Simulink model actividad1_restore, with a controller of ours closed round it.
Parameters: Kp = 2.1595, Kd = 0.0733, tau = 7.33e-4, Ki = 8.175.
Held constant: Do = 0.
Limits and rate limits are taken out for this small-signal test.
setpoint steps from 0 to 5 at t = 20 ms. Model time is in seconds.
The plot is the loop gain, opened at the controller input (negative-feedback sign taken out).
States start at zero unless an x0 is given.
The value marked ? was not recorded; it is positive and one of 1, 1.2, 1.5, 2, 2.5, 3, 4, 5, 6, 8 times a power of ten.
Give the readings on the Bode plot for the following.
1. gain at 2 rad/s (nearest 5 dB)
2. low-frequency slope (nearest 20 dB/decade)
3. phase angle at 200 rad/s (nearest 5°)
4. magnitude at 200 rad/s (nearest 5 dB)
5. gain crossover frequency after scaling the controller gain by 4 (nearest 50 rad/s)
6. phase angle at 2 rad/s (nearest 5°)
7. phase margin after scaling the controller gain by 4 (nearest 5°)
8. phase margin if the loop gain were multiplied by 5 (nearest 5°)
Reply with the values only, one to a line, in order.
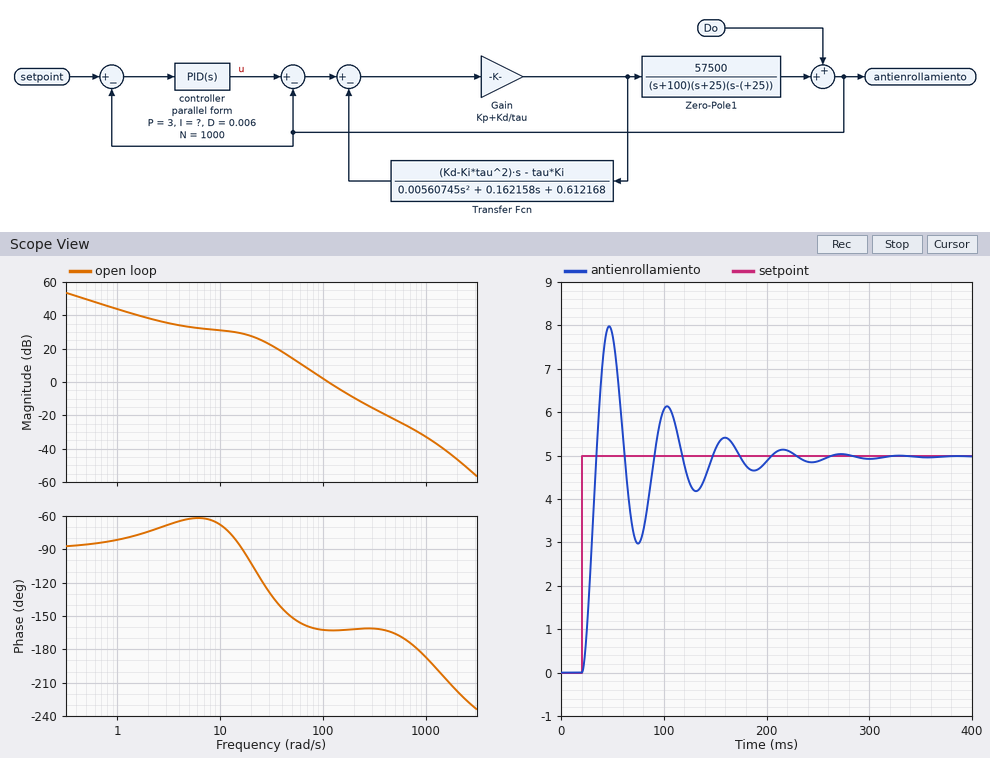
40 dB
-20 dB/decade
-160°
-10 dB
250 rad/s
-75°
20°
20°
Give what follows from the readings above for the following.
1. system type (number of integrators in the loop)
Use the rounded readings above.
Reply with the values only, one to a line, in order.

1
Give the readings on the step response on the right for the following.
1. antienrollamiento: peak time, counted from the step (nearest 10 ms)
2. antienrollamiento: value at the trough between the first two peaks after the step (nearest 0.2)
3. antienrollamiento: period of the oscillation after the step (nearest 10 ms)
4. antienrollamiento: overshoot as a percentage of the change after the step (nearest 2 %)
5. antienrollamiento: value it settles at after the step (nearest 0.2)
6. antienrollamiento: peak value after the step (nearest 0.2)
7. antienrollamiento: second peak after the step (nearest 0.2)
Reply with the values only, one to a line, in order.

30 ms
3.0
60 ms
60 %
5.0
8.0
6.2
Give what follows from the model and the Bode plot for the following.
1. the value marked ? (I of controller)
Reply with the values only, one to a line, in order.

150
